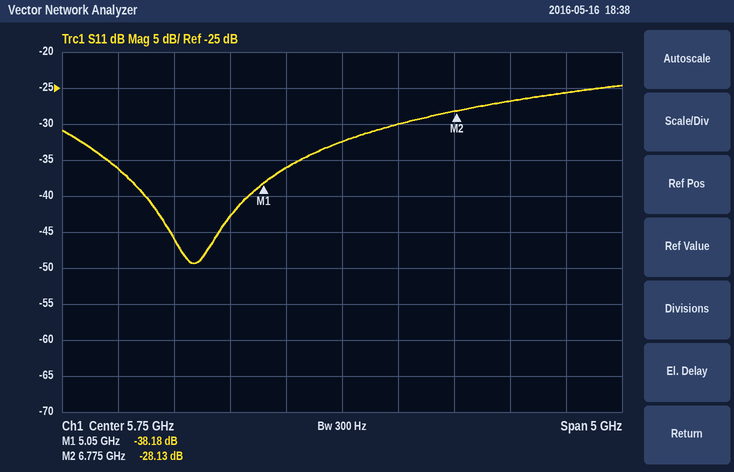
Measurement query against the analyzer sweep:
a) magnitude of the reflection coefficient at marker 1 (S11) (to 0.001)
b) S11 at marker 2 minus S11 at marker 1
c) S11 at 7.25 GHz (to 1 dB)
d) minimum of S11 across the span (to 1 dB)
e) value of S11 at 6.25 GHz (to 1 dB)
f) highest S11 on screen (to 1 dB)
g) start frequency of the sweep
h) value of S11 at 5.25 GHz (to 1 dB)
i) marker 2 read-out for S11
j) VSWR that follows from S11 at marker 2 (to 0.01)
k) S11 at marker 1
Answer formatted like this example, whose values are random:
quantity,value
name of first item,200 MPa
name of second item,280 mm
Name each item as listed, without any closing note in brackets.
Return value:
quantity,value
magnitude of the reflection coefficient at marker 1 (S11),0.012
S11 at marker 2 minus S11 at marker 1,10.05 dB
S11 at 7.25 GHz,-27 dB
minimum of S11 across the span,-49 dB
value of S11 at 6.25 GHz,-30 dB
highest S11 on screen,-25 dB
start frequency of the sweep,3.25 GHz
value of S11 at 5.25 GHz,-36 dB
marker 2 read-out for S11,-28.13 dB
VSWR that follows from S11 at marker 2,1.08
S11 at marker 1,-38.18 dB
